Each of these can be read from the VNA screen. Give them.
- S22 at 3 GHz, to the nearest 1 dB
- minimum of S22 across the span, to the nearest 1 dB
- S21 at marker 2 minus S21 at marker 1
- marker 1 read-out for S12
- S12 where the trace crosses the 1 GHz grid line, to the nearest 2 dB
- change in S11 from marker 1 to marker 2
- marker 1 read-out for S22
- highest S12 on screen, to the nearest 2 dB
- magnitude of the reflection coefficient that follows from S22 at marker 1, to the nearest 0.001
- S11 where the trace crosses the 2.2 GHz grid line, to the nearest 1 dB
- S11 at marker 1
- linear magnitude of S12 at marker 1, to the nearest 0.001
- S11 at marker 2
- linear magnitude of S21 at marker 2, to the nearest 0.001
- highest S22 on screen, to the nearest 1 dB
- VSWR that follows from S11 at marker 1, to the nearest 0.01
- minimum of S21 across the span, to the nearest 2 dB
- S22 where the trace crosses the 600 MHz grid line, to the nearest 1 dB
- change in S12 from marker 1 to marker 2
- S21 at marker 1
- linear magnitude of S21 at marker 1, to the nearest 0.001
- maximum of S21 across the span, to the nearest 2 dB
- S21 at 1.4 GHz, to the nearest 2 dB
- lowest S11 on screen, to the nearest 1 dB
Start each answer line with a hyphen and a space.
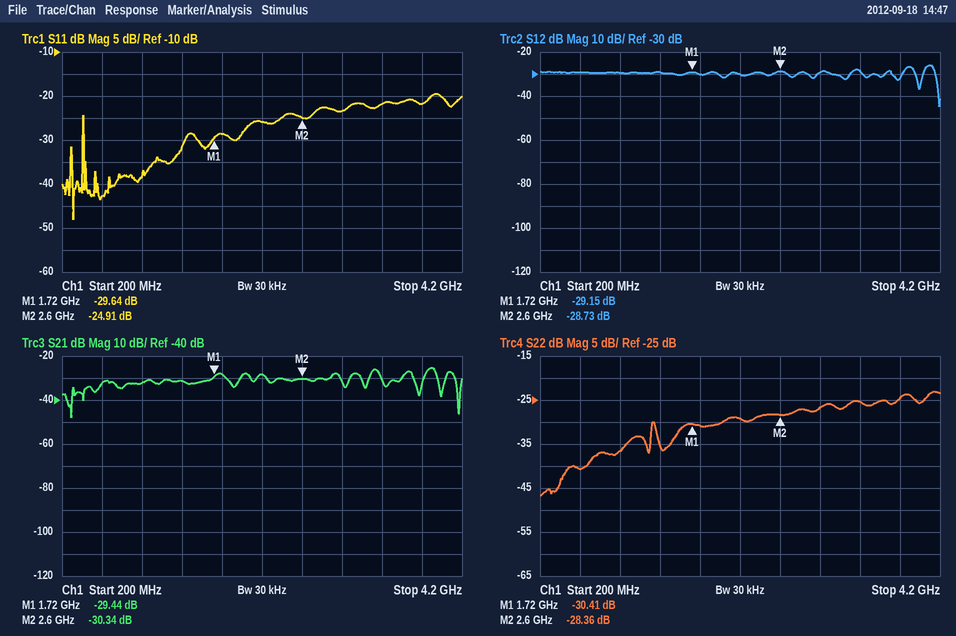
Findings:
- -27 dB
- -47 dB
- -0.90 dB
- -29.15 dB
- -30 dB
- 4.73 dB
- -30.41 dB
- -26 dB
- 0.030
- -26 dB
- -29.64 dB
- 0.035
- -24.91 dB
- 0.030
- -23 dB
- 1.07
- -48 dB
- -41 dB
- 0.42 dB
- -29.44 dB
- 0.034
- -26 dB
- -32 dB
- -48 dB
